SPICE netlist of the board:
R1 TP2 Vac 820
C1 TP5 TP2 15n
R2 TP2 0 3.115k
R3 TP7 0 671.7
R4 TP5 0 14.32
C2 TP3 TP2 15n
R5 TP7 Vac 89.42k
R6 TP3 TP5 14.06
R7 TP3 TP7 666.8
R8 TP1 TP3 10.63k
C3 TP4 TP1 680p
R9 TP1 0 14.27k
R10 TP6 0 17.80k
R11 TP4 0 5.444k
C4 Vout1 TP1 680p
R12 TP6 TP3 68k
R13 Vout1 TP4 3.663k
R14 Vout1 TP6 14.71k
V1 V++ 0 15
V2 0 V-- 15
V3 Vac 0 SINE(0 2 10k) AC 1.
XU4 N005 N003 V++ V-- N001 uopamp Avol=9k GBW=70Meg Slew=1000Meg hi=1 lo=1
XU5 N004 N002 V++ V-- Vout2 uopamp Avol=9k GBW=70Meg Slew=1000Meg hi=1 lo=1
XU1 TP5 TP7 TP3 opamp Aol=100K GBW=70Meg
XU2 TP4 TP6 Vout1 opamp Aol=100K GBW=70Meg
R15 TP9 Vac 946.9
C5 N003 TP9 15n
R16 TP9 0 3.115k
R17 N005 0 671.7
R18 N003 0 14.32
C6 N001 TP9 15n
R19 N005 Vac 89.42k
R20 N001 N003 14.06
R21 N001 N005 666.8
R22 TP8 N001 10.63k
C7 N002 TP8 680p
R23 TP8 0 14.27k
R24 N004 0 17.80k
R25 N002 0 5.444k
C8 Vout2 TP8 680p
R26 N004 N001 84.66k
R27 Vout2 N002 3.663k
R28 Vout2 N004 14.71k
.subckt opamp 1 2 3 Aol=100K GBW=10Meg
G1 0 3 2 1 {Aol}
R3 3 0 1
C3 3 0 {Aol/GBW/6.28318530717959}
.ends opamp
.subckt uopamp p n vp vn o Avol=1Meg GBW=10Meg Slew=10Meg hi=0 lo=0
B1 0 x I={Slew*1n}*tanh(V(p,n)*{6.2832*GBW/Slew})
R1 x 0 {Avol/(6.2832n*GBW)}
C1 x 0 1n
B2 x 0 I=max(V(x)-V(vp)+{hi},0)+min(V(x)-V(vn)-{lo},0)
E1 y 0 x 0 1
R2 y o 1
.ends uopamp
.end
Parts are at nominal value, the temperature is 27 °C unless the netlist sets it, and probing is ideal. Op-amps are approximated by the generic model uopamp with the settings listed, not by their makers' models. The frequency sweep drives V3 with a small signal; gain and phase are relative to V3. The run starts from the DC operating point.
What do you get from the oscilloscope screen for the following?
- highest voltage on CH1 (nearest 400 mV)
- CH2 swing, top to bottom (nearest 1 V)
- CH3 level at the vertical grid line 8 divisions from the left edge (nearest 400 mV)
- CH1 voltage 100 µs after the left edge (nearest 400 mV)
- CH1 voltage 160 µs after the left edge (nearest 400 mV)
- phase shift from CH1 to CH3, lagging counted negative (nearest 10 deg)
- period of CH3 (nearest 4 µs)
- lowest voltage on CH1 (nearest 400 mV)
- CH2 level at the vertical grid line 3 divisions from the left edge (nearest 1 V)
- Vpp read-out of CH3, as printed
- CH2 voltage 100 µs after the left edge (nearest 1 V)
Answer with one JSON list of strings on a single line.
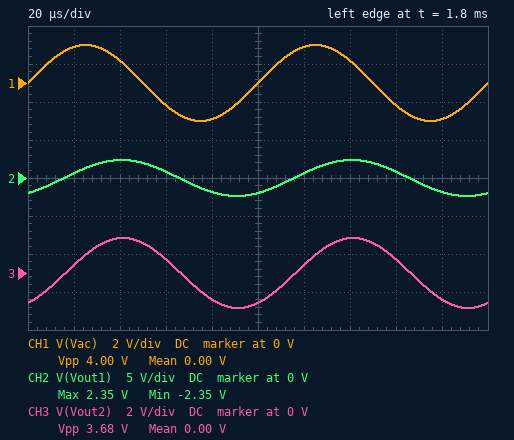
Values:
["2.0 V", "5 V", "800 mV", "0 V", "-1.2 V", "-60 deg", "100 µs", "-2.0 V", "1 V", "3.68 V", "-2 V"]
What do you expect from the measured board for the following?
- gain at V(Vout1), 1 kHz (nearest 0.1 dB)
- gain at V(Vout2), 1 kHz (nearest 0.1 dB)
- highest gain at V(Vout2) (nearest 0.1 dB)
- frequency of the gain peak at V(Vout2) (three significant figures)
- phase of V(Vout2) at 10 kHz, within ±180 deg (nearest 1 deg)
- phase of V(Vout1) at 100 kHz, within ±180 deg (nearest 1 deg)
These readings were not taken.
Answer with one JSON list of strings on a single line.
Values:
["-2.0 dB", "-3.1 dB", "1.5 dB", "27.8 kHz", "-59 deg", "82 deg"]
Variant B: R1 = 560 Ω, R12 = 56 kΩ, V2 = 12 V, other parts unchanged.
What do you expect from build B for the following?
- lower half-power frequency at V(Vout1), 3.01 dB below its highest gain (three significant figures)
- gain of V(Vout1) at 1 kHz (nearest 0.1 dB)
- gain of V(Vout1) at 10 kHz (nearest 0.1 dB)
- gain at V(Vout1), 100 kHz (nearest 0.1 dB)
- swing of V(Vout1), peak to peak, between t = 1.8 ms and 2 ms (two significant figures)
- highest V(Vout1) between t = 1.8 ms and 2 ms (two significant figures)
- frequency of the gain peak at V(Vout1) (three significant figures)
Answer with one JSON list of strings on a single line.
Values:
["14.2 kHz", "-1.4 dB", "4.1 dB", "-28.6 dB", "6.4 V", "3.2 V", "17.0 kHz"]
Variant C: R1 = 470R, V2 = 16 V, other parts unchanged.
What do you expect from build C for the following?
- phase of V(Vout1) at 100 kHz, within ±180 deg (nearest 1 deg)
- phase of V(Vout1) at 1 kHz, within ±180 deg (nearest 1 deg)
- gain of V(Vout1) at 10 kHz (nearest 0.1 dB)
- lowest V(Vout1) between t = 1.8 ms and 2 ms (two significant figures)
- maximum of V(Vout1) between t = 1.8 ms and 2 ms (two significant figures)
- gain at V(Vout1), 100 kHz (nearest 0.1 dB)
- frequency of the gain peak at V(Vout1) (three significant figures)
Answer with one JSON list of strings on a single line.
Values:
["65 deg", "-5 deg", "3.9 dB", "-3.1 V", "3.1 V", "-28.9 dB", "18.3 kHz"]
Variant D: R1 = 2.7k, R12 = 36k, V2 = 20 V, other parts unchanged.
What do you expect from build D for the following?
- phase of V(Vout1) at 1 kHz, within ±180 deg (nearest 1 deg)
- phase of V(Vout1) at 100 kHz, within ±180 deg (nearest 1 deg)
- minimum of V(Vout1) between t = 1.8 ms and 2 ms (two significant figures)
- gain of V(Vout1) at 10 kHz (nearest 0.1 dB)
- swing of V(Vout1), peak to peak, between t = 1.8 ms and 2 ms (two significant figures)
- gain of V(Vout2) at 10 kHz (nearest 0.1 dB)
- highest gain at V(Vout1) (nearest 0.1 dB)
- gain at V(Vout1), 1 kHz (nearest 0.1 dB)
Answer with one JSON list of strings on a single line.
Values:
["-1 deg", "-129 deg", "-2.1 V", "0.5 dB", "4.3 V", "-0.7 dB", "0.7 dB", "-0.1 dB"]
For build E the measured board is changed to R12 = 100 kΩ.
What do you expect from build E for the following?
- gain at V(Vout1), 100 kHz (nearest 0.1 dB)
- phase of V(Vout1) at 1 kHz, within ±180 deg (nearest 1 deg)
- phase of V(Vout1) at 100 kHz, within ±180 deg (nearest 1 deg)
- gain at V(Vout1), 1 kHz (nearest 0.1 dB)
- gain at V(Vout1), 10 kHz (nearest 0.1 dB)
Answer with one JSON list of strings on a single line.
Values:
["-47.9 dB", "-5 deg", "150 deg", "-3.6 dB", "0.1 dB"]
